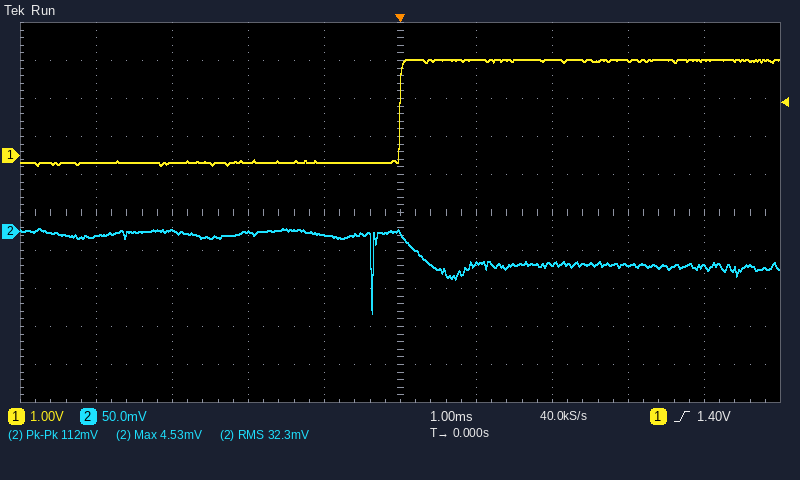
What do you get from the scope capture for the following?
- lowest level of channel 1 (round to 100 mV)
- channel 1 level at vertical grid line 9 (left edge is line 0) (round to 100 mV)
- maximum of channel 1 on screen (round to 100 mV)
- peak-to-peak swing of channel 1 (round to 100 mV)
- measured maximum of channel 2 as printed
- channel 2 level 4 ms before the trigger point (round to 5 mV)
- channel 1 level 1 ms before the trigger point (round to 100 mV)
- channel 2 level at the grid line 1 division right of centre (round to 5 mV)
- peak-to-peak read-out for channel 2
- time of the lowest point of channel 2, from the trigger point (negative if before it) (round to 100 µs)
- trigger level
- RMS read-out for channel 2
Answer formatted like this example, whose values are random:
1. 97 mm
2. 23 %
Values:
1. -300 mV
2. 2.5 V
3. 2.5 V
4. 2.8 V
5. 4.53 mV
6. -5 mV
7. -200 mV
8. -45 mV
9. 112 mV
10. -400 µs
11. 1.40 V
12. 32.3 mV
